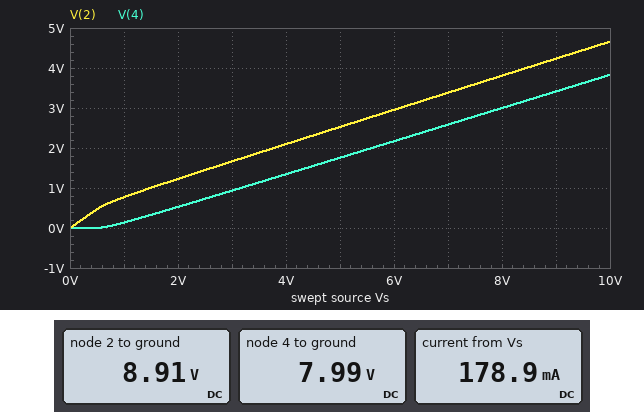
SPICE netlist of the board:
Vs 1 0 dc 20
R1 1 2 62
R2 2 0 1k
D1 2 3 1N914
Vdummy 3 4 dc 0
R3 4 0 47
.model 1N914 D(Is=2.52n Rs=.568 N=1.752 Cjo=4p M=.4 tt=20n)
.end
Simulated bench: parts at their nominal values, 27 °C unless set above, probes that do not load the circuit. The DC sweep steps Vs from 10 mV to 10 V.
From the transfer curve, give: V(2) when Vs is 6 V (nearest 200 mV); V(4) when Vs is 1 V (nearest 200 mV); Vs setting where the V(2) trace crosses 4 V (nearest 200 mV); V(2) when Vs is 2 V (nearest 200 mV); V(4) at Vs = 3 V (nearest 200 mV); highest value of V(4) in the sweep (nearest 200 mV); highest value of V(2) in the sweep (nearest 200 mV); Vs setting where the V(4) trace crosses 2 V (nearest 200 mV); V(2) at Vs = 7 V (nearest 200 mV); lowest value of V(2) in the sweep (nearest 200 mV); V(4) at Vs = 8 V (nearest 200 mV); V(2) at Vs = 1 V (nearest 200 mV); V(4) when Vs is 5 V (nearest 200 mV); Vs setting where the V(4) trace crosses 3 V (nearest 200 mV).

3.0 V
200 mV
8.4 V
1.2 V
1.0 V
3.8 V
4.6 V
5.6 V
3.4 V
0 V
3.0 V
800 mV
1.8 V
8.0 V
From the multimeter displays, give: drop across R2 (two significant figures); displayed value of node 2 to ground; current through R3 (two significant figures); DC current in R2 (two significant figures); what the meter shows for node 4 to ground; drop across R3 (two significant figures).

8.9 V
8.91 V
170 mA
8.9 mA
7.99 V
8.0 V
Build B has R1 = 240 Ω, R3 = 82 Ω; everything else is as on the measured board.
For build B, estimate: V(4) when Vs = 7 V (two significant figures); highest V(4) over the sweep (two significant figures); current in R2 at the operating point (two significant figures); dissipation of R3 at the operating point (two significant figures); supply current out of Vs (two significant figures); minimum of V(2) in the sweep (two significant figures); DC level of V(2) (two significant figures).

1.5 V
2.2 V
5.4 mA
250 mW
61 mA
8.1 mV
5.4 V
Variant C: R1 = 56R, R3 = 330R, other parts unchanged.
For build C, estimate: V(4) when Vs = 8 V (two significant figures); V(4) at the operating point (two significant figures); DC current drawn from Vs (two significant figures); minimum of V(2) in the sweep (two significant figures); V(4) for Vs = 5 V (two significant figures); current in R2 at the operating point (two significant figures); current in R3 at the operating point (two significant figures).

5.9 V
16 V
64 mA
9.5 mV
3.5 V
16 mA
47 mA
